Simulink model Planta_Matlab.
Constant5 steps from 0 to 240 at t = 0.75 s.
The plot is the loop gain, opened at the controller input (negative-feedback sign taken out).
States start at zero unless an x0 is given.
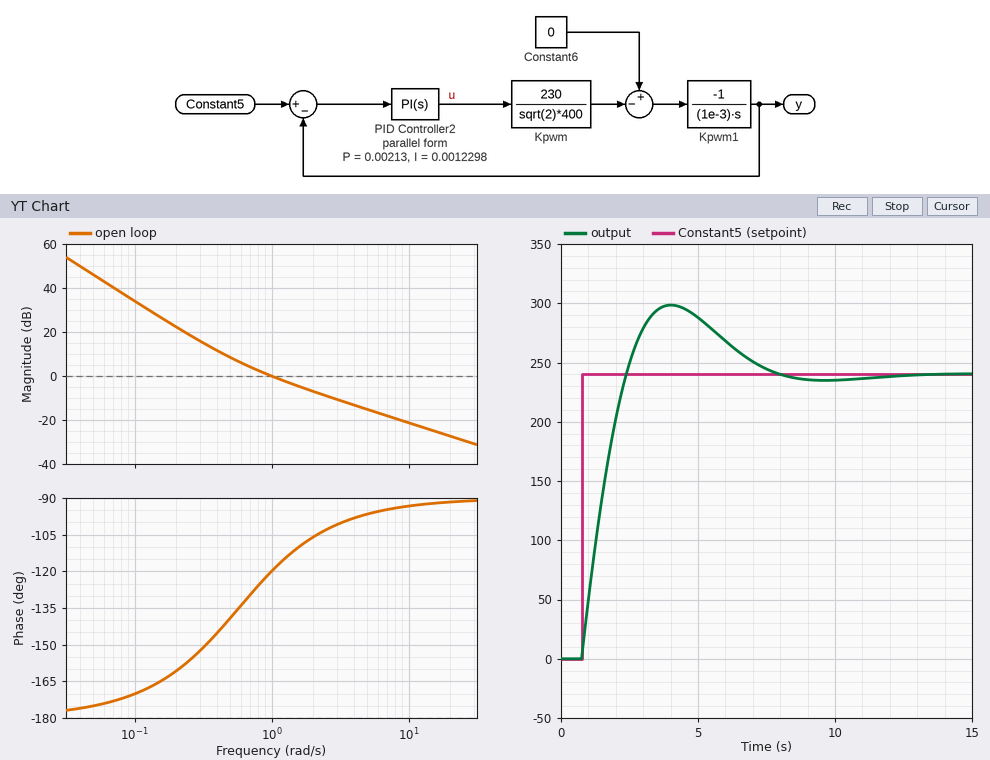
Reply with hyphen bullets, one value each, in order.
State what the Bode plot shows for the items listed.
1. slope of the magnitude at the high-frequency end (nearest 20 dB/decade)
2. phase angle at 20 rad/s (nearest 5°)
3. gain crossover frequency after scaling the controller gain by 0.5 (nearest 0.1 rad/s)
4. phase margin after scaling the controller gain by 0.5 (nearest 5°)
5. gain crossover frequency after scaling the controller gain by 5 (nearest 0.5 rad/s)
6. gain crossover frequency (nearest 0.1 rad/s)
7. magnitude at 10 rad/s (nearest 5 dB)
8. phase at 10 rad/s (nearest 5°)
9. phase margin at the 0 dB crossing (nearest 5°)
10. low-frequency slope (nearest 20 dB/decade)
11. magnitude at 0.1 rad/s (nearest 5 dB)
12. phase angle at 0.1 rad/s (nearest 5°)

- -20 dB/decade
- -90°
- 0.6 rad/s
- 45°
- 4.5 rad/s
- 1.0 rad/s
- -20 dB
- -95°
- 60°
- -40 dB/decade
- 35 dB
- -170°
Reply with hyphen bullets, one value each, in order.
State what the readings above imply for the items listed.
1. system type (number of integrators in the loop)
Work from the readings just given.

- 2
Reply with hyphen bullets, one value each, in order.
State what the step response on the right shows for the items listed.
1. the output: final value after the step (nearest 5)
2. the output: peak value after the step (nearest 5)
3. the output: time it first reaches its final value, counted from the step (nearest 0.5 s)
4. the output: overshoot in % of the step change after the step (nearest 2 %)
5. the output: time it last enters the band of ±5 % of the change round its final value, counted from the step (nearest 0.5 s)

- 240
- 300
- 1.5 s
- 24 %
- 6.0 s
